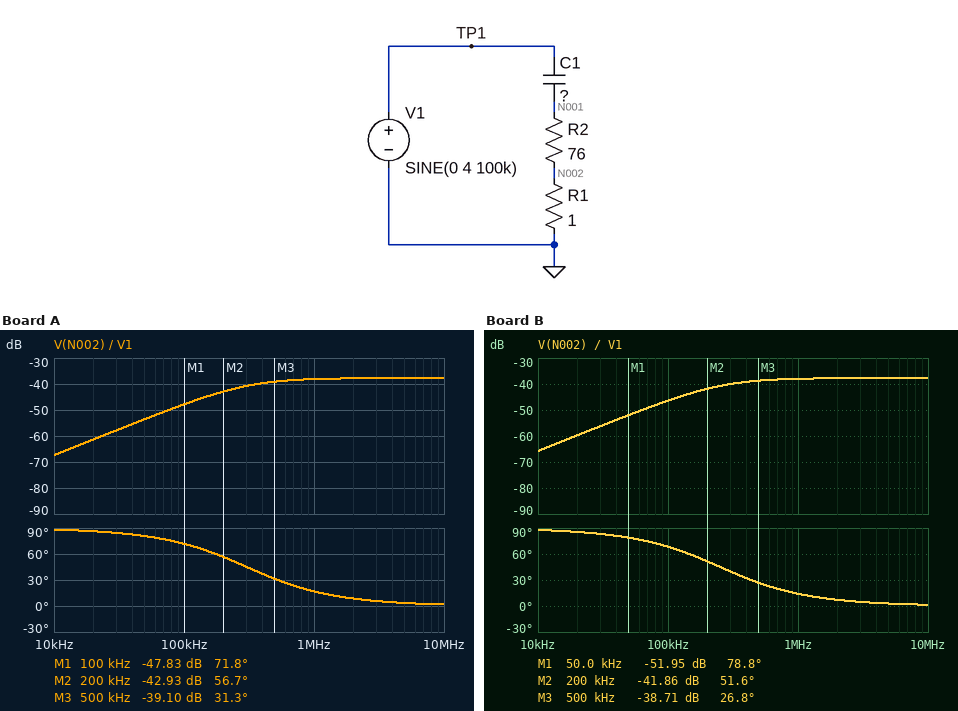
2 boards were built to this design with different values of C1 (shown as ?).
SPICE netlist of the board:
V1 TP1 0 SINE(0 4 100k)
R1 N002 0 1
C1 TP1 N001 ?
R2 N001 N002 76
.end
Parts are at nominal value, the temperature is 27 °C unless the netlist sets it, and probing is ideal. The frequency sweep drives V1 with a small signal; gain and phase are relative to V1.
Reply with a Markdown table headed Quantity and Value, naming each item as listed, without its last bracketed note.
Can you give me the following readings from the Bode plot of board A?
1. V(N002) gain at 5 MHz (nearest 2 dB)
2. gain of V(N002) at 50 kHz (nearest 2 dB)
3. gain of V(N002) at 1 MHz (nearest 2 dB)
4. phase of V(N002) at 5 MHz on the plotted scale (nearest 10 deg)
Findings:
| Quantity | Value |
|---|---|
| V(N002) gain at 5 MHz | -38 dB |
| gain of V(N002) at 50 kHz | -54 dB |
| gain of V(N002) at 1 MHz | -38 dB |
| phase of V(N002) at 5 MHz on the plotted scale | 0 deg |
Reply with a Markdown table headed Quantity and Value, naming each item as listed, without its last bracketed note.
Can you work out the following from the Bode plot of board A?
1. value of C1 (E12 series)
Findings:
| Quantity | Value |
|---|---|
| value of C1 | 6.8 nF |
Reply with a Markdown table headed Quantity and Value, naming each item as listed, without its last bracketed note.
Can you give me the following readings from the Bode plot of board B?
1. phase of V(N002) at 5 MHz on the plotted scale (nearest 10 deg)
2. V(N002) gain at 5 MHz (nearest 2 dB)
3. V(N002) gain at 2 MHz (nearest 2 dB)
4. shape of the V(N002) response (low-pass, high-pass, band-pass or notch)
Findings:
| Quantity | Value |
|---|---|
| phase of V(N002) at 5 MHz on the plotted scale | 0 deg |
| V(N002) gain at 5 MHz | -38 dB |
| V(N002) gain at 2 MHz | -38 dB |
| shape of the V(N002) response | high-pass |
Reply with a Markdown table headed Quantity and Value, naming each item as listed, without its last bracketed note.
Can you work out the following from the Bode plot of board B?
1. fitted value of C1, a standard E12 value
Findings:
| Quantity | Value |
|---|---|
| fitted value of C1, a standard E12 value | 8.2 nF |
